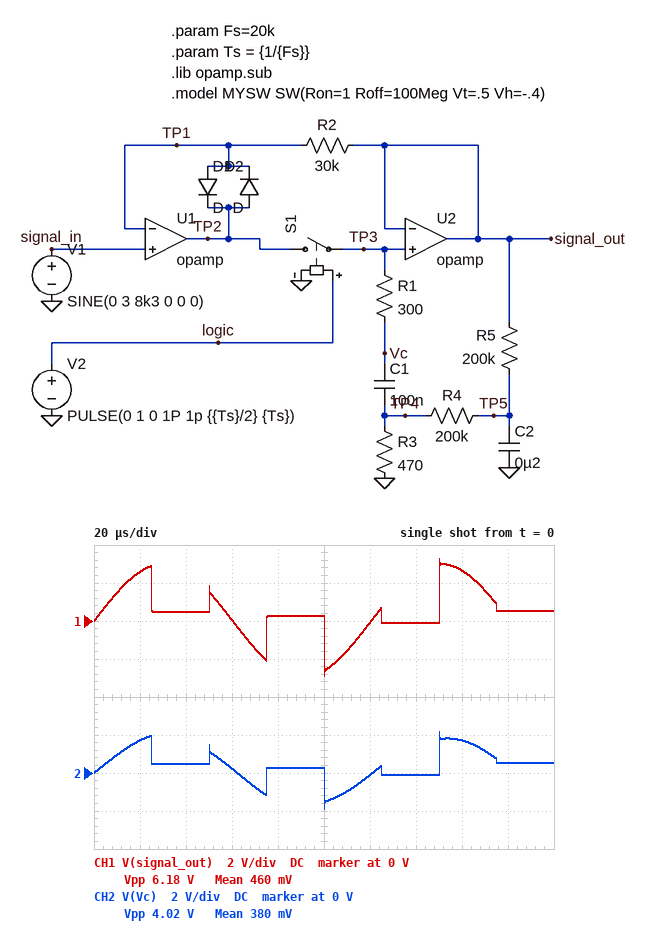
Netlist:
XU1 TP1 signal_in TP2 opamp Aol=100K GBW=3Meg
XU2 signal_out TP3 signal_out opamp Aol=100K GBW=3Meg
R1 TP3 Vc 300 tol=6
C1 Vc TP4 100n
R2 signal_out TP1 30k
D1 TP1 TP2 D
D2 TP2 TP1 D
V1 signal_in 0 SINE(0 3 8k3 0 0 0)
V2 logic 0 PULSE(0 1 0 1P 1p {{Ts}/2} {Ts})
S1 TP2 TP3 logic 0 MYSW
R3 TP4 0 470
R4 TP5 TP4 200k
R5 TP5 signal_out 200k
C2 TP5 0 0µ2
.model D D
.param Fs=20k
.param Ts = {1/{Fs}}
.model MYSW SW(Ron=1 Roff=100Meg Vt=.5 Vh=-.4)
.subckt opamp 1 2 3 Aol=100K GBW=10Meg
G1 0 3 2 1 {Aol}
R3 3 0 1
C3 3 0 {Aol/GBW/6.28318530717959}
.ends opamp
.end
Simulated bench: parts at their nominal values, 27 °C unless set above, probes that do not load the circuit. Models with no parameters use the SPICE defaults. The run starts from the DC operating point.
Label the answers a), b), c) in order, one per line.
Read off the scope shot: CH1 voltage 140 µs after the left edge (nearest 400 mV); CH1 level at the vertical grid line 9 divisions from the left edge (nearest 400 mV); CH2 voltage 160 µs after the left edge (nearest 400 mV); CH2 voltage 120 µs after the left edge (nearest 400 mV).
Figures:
a) 0 V
b) 400 mV
c) 1.6 V
d) 0 V
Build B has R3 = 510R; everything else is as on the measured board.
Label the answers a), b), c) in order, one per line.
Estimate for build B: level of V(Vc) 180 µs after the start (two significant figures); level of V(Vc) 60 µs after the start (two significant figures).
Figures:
a) 510 mV
b) 210 mV
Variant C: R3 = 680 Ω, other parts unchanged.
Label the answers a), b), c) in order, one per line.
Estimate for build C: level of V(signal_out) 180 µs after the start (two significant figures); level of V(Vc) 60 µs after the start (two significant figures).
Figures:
a) 450 mV
b) 160 mV
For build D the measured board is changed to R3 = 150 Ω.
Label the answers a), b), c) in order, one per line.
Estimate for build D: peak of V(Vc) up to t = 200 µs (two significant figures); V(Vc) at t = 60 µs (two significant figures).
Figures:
a) 1.5 V
b) 530 mV
